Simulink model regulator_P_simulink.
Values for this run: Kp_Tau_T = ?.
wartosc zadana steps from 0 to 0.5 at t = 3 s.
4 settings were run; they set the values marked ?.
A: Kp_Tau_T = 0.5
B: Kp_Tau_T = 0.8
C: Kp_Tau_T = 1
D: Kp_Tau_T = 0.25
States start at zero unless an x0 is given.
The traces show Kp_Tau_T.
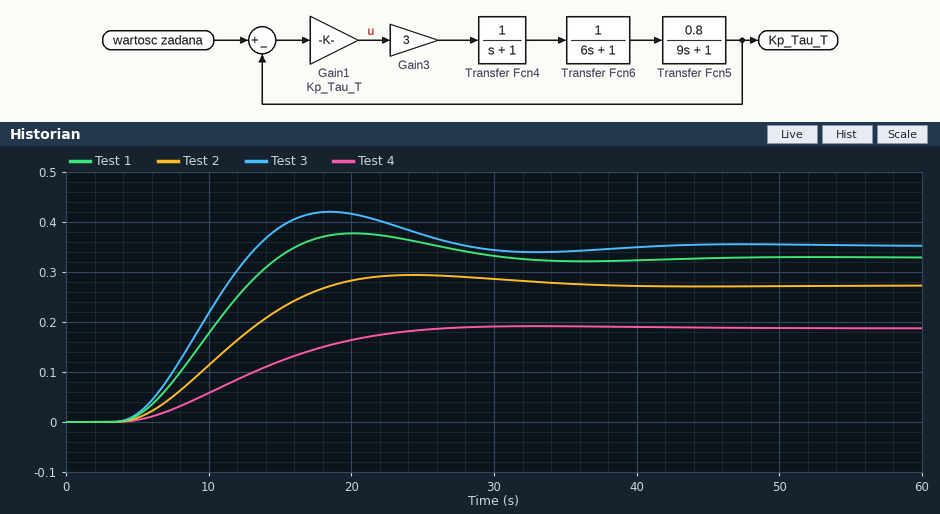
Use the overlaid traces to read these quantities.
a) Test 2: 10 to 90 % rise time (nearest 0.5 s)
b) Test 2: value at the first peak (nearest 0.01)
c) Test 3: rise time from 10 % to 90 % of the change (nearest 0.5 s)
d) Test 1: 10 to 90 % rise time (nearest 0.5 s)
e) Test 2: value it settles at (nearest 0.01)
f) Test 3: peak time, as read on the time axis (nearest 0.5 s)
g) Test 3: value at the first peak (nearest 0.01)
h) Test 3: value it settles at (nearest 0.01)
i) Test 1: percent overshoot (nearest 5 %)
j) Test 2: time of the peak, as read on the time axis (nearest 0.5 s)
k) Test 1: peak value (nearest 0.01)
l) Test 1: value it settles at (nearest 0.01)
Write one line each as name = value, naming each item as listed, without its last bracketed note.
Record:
Test 2: 10 to 90 % rise time = 10.0 s
Test 2: value at the first peak = 0.29
Test 3: rise time from 10 % to 90 % of the change = 6.5 s
Test 1: 10 to 90 % rise time = 7.5 s
Test 2: value it settles at = 0.27
Test 3: peak time, as read on the time axis = 18.5 s
Test 3: value at the first peak = 0.42
Test 3: value it settles at = 0.35
Test 1: percent overshoot = 15 %
Test 2: time of the peak, as read on the time axis = 24.5 s
Test 1: peak value = 0.38
Test 1: value it settles at = 0.33
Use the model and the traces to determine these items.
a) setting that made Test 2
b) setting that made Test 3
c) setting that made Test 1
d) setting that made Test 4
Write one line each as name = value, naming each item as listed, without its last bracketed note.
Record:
setting that made Test 2 = A
setting that made Test 3 = C
setting that made Test 1 = B
setting that made Test 4 = D
